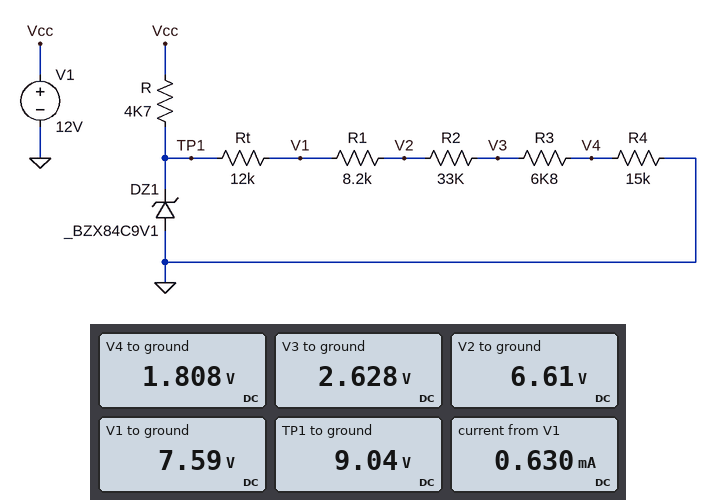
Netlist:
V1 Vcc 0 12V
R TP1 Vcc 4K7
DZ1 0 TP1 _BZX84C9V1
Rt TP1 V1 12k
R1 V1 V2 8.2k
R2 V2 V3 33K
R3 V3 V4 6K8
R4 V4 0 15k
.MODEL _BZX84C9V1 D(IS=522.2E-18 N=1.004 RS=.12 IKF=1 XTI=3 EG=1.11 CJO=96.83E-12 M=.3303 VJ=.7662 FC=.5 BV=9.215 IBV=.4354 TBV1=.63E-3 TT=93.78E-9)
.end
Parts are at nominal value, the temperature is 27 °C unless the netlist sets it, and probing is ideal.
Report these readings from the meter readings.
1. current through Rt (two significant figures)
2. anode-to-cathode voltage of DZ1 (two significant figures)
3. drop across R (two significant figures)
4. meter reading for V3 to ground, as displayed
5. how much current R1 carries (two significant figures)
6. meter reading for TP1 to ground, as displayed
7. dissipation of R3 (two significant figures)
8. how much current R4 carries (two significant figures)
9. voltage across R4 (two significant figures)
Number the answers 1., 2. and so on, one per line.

1. 120 µA
2. -9.0 V
3. 3.0 V
4. 2.628 V
5. 120 µA
6. 9.04 V
7. 99 µW
8. 120 µA
9. 1.8 V
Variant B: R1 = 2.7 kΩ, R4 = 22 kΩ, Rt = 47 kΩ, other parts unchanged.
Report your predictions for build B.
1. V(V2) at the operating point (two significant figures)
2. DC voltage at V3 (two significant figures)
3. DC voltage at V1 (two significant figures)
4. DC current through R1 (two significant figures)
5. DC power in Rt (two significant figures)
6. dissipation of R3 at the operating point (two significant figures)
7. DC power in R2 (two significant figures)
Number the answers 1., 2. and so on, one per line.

1. 5.0 V
2. 2.3 V
3. 5.2 V
4. 81 µA
5. 310 µW
6. 45 µW
7. 220 µW
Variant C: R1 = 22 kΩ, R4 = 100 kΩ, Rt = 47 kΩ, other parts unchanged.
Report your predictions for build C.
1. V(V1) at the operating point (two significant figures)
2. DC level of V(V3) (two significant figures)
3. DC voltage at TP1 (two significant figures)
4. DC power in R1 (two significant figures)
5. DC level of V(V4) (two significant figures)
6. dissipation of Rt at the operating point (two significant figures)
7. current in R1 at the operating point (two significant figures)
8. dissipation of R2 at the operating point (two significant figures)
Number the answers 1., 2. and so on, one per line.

1. 7.0 V
2. 4.6 V
3. 9.0 V
4. 41 µW
5. 4.3 V
6. 88 µW
7. 43 µA
8. 62 µW
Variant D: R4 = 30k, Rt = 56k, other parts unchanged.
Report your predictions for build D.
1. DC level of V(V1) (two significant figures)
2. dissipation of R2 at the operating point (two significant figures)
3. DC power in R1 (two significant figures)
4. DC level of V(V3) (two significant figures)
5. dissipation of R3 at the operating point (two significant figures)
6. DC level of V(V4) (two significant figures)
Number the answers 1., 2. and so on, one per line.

1. 5.3 V
2. 150 µW
3. 37 µW
4. 2.5 V
5. 31 µW
6. 2.0 V
